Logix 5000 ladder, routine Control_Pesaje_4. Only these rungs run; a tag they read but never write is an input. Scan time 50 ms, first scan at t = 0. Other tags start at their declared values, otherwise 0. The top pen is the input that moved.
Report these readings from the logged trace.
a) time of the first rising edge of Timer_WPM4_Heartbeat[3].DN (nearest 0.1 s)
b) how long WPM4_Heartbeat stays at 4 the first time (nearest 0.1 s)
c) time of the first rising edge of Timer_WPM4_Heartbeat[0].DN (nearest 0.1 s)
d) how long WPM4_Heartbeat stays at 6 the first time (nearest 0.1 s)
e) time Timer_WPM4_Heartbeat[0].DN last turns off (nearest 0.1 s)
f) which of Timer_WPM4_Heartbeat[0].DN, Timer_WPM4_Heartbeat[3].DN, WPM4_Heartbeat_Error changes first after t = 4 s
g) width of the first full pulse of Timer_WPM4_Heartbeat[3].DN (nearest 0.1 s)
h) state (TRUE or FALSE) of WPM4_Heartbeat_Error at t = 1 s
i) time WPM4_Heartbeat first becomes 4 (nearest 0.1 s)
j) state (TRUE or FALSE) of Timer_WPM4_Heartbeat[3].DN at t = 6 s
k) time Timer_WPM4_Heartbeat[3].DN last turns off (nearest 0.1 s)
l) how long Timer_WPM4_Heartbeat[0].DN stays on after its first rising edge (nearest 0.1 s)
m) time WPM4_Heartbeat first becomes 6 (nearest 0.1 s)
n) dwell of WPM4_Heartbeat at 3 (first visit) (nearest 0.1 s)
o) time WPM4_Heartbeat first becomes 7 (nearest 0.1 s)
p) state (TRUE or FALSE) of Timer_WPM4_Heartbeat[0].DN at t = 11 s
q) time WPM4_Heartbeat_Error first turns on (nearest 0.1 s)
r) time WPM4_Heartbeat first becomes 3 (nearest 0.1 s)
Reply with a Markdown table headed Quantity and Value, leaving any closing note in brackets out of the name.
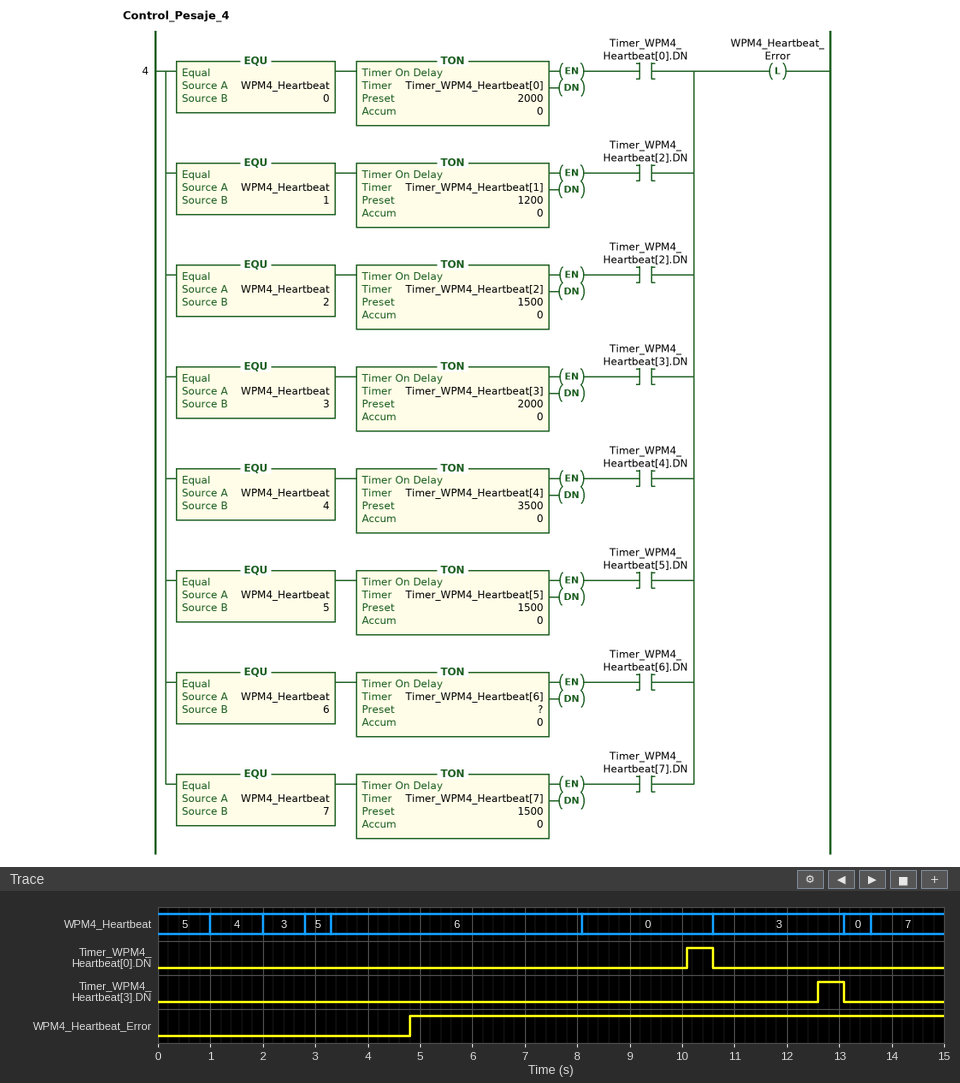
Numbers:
| Quantity | Value |
|---|---|
| time of the first rising edge of Timer_WPM4_Heartbeat[3].DN | 12.6 s |
| how long WPM4_Heartbeat stays at 4 the first time | 1.0 s |
| time of the first rising edge of Timer_WPM4_Heartbeat[0].DN | 10.1 s |
| how long WPM4_Heartbeat stays at 6 the first time | 4.8 s |
| time Timer_WPM4_Heartbeat[0].DN last turns off | 10.6 s |
| which of Timer_WPM4_Heartbeat[0].DN, Timer_WPM4_Heartbeat[3].DN, WPM4_Heartbeat_Error changes first after t = 4 s | WPM4_Heartbeat_Error |
| width of the first full pulse of Timer_WPM4_Heartbeat[3].DN | 0.5 s |
| state (TRUE or FALSE) of WPM4_Heartbeat_Error at t = 1 s | FALSE |
| time WPM4_Heartbeat first becomes 4 | 1.0 s |
| state (TRUE or FALSE) of Timer_WPM4_Heartbeat[3].DN at t = 6 s | FALSE |
| time Timer_WPM4_Heartbeat[3].DN last turns off | 13.1 s |
| how long Timer_WPM4_Heartbeat[0].DN stays on after its first rising edge | 0.5 s |
| time WPM4_Heartbeat first becomes 6 | 3.3 s |
| dwell of WPM4_Heartbeat at 3 (first visit) | 0.8 s |
| time WPM4_Heartbeat first becomes 7 | 13.6 s |
| state (TRUE or FALSE) of Timer_WPM4_Heartbeat[0].DN at t = 11 s | FALSE |
| time WPM4_Heartbeat_Error first turns on | 4.8 s |
| time WPM4_Heartbeat first becomes 3 | 2.0 s |
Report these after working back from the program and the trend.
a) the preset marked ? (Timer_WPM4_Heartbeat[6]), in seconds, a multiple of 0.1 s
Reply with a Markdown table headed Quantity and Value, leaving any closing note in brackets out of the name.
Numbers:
| Quantity | Value |
|---|---|
| the preset marked ? (Timer_WPM4_Heartbeat[6]), in seconds, a multiple of 0.1 s | 1.5 s |
